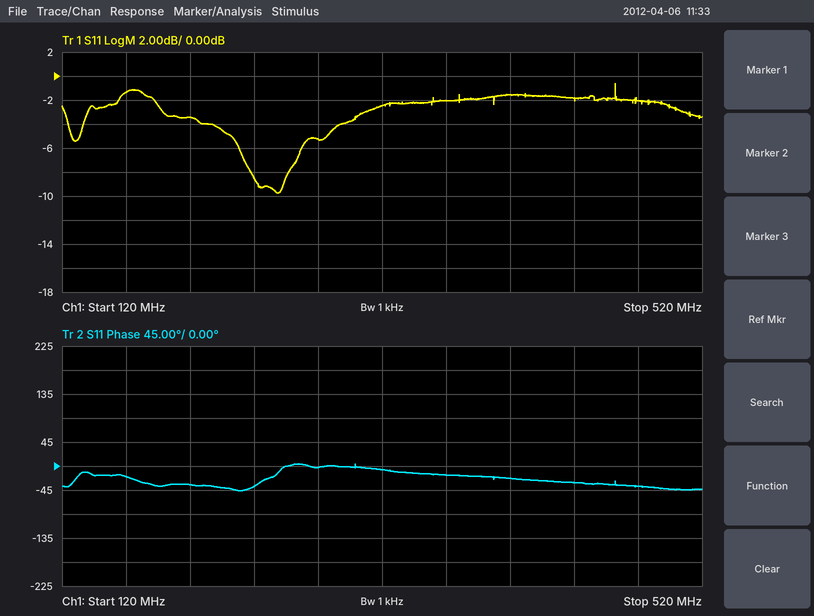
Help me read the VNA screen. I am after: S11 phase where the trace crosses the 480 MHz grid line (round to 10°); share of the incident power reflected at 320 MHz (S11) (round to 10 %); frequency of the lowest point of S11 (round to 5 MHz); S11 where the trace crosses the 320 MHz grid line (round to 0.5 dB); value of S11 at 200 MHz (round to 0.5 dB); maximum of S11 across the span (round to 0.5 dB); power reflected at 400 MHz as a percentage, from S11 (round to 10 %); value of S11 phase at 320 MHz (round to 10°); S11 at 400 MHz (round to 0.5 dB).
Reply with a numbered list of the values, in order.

1. -40°
2. 60 %
3. 255 MHz
4. -2.5 dB
5. -3.5 dB
6. -0.5 dB
7. 70 %
8. -10°
9. -1.5 dB
